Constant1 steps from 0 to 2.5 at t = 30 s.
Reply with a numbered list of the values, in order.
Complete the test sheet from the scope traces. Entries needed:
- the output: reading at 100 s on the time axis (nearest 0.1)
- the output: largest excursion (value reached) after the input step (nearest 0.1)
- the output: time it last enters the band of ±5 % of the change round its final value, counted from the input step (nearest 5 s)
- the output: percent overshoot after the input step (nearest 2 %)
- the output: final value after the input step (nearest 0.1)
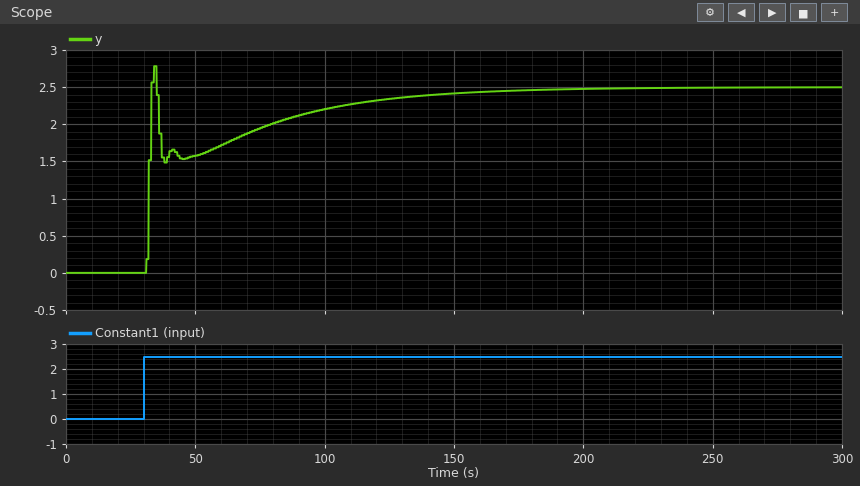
1. 2.2
2. 2.8
3. 105 s
4. 12 %
5. 2.5
